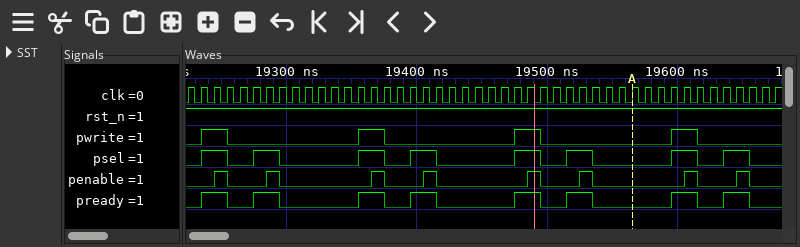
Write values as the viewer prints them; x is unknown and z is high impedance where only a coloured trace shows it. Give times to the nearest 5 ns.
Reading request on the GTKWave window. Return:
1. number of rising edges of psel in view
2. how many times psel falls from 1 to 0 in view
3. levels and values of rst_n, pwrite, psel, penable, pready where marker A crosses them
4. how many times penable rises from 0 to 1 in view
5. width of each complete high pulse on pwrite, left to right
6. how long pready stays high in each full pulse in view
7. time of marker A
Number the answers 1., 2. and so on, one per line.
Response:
1. 8
2. 8
3. rst_n=1, pwrite=0, psel=0, penable=0, pready=0
4. 8
5. 20 ns, 20 ns, 20 ns, 20 ns
6. 20 ns, 20 ns, 20 ns, 20 ns, 20 ns, 20 ns, 20 ns, 20 ns
7. 19565 ns
